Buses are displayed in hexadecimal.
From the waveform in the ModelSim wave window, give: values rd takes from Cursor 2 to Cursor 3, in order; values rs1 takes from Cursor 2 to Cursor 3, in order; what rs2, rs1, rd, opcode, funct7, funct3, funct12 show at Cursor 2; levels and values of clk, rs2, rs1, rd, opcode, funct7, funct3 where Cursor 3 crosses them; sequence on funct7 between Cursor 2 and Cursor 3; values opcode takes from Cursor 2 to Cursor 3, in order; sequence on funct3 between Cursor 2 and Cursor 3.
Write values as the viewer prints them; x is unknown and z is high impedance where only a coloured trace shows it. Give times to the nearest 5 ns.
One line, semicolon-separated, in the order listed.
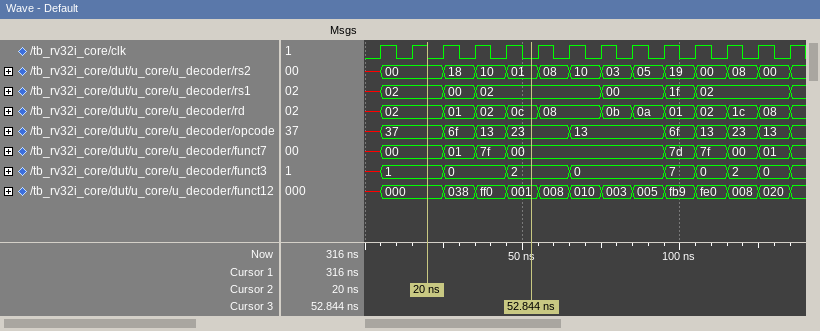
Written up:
02, 01, 02, 0c; 02, 00, 02; rs2=00, rs1=02, rd=02, opcode=37, funct7=00, funct3=1, funct12=000; clk=0, rs2=01, rs1=02, rd=0c, opcode=23, funct7=00, funct3=2; 00, 01, 7f, 00; 37, 6f, 13, 23; 1, 0, 2
